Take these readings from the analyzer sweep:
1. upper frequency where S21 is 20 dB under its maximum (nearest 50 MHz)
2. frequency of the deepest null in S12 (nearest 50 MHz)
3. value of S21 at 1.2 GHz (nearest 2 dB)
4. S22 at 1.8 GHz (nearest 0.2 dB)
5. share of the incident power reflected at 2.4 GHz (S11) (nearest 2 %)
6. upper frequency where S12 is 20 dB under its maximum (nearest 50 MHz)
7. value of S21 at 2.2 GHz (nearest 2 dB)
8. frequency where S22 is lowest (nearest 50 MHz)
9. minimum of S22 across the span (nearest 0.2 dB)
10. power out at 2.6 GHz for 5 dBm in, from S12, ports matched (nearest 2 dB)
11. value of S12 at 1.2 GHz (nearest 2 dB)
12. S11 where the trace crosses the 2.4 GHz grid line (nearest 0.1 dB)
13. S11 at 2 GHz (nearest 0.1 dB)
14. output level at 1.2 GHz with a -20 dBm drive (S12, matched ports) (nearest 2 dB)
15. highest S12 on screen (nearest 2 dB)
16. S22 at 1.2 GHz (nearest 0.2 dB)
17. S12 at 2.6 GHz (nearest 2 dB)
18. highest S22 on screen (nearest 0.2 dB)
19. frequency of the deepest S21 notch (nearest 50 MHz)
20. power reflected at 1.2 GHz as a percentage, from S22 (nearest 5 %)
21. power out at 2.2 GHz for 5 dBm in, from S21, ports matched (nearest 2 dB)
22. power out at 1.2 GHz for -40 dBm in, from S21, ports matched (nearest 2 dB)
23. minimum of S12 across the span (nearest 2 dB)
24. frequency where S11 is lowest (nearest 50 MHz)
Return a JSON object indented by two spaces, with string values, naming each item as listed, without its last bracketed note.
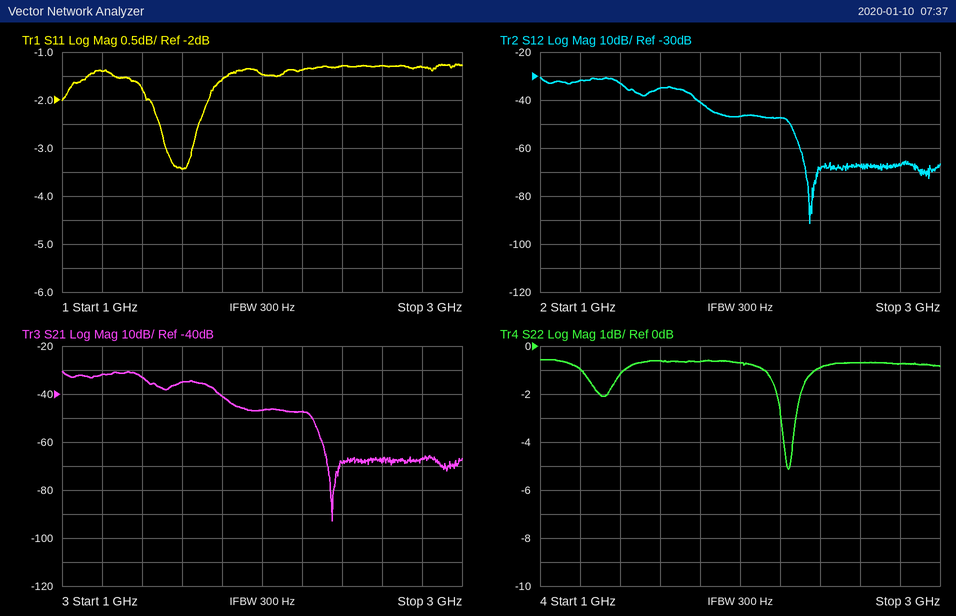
{
  "upper frequency where S21 is 20 dB under its maximum": "2.25 GHz",
  "frequency of the deepest null in S12": "2.35 GHz",
  "value of S21 at 1.2 GHz": "-32 dB",
  "S22 at 1.8 GHz": "-0.6 dB",
  "share of the incident power reflected at 2.4 GHz (S11)": "74 %",
  "upper frequency where S12 is 20 dB under its maximum": "2.25 GHz",
  "value of S21 at 2.2 GHz": "-48 dB",
  "frequency where S22 is lowest": "2.25 GHz",
  "minimum of S22 across the span": "-5.2 dB",
  "power out at 2.6 GHz for 5 dBm in, from S12, ports matched": "-62 dBm",
  "value of S12 at 1.2 GHz": "-32 dB",
  "S11 where the trace crosses the 2.4 GHz grid line": "-1.3 dB",
  "S11 at 2 GHz": "-1.5 dB",
  "output level at 1.2 GHz with a -20 dBm drive (S12, matched ports)": "-52 dBm",
  "highest S12 on screen": "-30 dB",
  "S22 at 1.2 GHz": "-1.0 dB",
  "S12 at 2.6 GHz": "-68 dB",
  "highest S22 on screen": "-0.6 dB",
  "frequency of the deepest S21 notch": "2.35 GHz",
  "power reflected at 1.2 GHz as a percentage, from S22": "80 %",
  "power out at 2.2 GHz for 5 dBm in, from S21, ports matched": "-42 dBm",
  "power out at 1.2 GHz for -40 dBm in, from S21, ports matched": "-72 dBm",
  "minimum of S12 across the span": "-92 dB",
  "frequency where S11 is lowest": "1.60 GHz"
}
